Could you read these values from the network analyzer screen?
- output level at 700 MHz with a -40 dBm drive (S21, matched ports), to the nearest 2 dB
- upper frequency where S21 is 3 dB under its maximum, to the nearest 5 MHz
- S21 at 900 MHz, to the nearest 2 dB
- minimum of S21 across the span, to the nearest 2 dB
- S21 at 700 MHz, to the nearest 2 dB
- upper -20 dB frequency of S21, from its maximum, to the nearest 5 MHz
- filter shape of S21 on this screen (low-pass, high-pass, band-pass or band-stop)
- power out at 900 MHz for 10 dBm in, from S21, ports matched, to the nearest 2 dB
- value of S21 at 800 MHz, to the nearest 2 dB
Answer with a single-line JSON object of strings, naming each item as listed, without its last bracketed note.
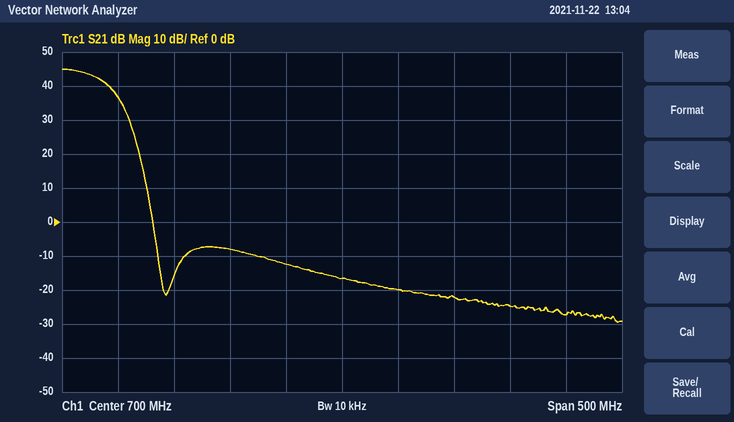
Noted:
{"output level at 700 MHz with a -40 dBm drive (S21, matched ports), to the nearest 2 dB": "-56 dBm", "upper frequency where S21 is 3 dB under its maximum, to the nearest 5 MHz": "485 MHz", "S21 at 900 MHz, to the nearest 2 dB": "-28 dB", "minimum of S21 across the span, to the nearest 2 dB": "-30 dB", "S21 at 700 MHz, to the nearest 2 dB": "-16 dB", "upper -20 dB frequency of S21, from its maximum, to the nearest 5 MHz": "515 MHz", "filter shape of S21 on this screen": "low-pass", "power out at 900 MHz for 10 dBm in, from S21, ports matched, to the nearest 2 dB": "-18 dBm", "value of S21 at 800 MHz, to the nearest 2 dB": "-22 dB"}
